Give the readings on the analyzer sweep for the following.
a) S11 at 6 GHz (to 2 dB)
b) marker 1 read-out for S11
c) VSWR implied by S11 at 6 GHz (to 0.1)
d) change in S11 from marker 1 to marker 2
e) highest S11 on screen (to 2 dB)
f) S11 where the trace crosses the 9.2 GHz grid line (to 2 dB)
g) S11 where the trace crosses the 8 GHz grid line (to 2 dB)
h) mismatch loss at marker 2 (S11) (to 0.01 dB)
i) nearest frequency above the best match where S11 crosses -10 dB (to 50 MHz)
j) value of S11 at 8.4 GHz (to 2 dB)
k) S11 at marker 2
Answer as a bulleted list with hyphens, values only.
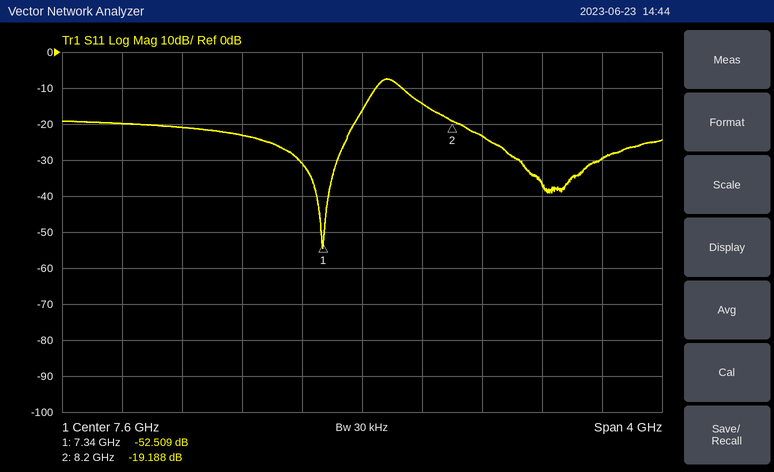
- -20 dB
- -52.509 dB
- 1.2
- 33.321 dB
- -8 dB
- -30 dB
- -14 dB
- 0.05 dB
- 7.70 GHz
- -24 dB
- -19.188 dB
